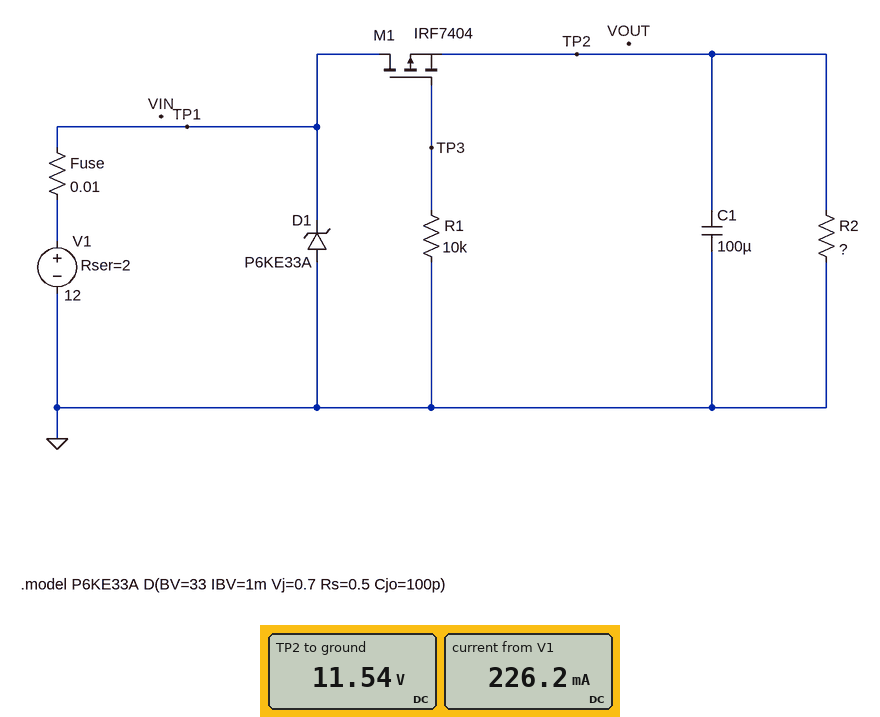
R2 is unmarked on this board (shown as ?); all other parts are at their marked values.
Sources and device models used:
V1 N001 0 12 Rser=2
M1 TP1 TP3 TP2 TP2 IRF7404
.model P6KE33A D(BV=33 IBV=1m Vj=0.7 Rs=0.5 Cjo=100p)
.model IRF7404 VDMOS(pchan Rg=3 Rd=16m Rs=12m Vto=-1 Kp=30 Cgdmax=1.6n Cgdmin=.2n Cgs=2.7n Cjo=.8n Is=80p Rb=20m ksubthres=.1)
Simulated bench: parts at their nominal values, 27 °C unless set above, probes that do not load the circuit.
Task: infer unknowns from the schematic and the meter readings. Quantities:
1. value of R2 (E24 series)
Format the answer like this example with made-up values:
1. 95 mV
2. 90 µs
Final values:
1. 51 Ω
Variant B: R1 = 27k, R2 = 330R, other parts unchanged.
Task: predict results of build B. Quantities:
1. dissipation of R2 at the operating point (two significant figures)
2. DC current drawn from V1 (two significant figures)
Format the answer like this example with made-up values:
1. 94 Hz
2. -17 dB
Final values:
1. 430 mW
2. 36 mA
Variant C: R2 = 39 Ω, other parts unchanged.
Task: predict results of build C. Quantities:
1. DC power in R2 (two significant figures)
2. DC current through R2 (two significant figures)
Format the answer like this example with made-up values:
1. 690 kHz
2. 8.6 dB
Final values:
1. 3.3 W
2. 290 mA
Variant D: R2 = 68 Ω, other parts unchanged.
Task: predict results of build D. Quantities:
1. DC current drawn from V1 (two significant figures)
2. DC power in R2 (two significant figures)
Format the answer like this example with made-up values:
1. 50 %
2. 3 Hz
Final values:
1. 170 mA
2. 2.0 W
